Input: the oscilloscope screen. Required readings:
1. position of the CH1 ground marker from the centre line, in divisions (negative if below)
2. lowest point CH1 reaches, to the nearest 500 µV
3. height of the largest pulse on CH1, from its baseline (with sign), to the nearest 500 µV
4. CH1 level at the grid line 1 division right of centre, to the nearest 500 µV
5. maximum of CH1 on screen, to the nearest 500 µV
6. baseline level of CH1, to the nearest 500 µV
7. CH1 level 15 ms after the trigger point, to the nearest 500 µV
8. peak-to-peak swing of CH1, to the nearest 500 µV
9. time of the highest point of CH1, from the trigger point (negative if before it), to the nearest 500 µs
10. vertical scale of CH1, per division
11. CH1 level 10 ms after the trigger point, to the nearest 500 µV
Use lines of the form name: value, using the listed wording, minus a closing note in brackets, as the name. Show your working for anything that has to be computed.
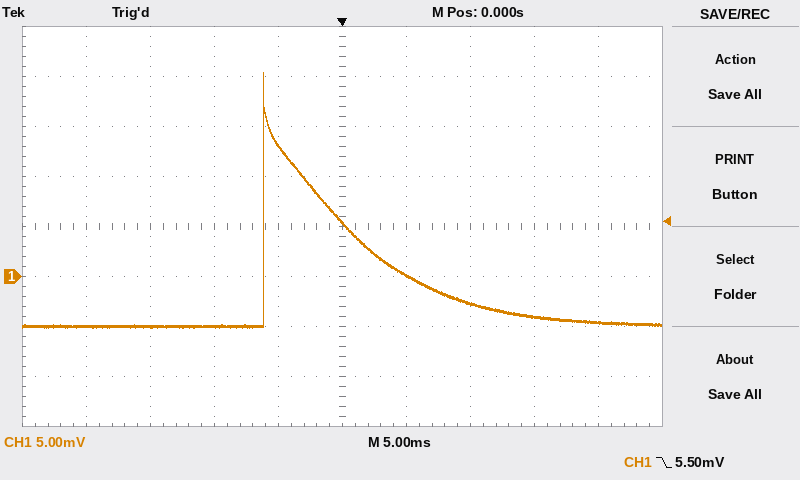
position of the CH1 ground marker from the centre line, in divisions: -1.0 div
lowest point CH1 reaches, to the nearest 500 µV: -5.0 mV
height of the largest pulse on CH1, from its baseline (with sign), to the nearest 500 µV: 20.5 mV − (-5.0 mV) = +25.5 mV
CH1 level at the grid line 1 division right of centre, to the nearest 500 µV: 0.0 mV
maximum of CH1 on screen, to the nearest 500 µV: 20.5 mV
baseline level of CH1, to the nearest 500 µV: -5.0 mV
CH1 level 15 ms after the trigger point, to the nearest 500 µV: -4.0 mV
peak-to-peak swing of CH1, to the nearest 500 µV: 20.5 mV − (-5.0 mV) = 25.5 mV
time of the highest point of CH1, from the trigger point (negative if before it), to the nearest 500 µs: -6.0 ms
vertical scale of CH1, per division: 5 mV
CH1 level 10 ms after the trigger point, to the nearest 500 µV: -2.5 mV
